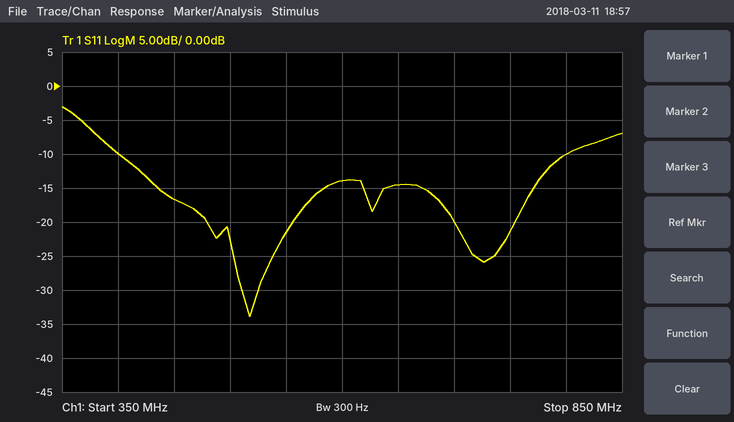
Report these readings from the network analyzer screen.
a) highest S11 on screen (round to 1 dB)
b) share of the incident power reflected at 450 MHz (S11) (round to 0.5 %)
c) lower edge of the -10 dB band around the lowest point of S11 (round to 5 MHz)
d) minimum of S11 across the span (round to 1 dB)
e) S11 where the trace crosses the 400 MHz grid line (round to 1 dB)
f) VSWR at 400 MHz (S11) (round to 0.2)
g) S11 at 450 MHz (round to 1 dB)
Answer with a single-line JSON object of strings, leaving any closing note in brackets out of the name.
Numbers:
{"highest S11 on screen": "-3 dB", "share of the incident power reflected at 450 MHz (S11)": "2.0 %", "lower edge of the -10 dB band around the lowest point of S11": "400 MHz", "minimum of S11 across the span": "-34 dB", "S11 where the trace crosses the 400 MHz grid line": "-10 dB", "VSWR at 400 MHz (S11)": "2.0", "S11 at 450 MHz": "-17 dB"}
